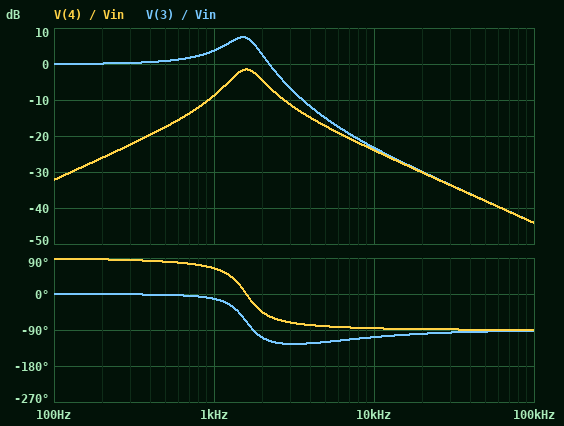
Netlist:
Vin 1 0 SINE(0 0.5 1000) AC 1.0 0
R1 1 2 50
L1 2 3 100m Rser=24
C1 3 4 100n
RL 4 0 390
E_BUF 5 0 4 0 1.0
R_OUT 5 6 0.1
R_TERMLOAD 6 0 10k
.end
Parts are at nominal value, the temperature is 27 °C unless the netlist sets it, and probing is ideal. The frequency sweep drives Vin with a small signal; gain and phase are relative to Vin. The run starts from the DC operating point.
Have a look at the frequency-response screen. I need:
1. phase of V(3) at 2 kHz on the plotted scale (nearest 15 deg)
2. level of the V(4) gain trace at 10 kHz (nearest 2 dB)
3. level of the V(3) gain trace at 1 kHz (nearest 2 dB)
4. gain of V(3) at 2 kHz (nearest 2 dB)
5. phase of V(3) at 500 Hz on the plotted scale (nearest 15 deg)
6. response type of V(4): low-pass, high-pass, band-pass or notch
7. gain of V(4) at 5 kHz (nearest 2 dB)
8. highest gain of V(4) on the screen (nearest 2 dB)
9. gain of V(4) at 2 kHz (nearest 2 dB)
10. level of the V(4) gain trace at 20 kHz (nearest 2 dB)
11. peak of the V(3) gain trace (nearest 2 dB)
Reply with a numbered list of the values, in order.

1. -105 deg
2. -24 dB
3. 4 dB
4. 2 dB
5. 0 deg
6. band-pass
7. -18 dB
8. -2 dB
9. -4 dB
10. -30 dB
11. 8 dB
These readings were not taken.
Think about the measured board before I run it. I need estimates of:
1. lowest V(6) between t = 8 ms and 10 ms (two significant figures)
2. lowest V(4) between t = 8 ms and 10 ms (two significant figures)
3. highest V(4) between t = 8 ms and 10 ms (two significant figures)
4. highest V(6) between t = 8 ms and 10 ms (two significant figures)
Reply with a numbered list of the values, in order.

1. -180 mV
2. -180 mV
3. 180 mV
4. 180 mV
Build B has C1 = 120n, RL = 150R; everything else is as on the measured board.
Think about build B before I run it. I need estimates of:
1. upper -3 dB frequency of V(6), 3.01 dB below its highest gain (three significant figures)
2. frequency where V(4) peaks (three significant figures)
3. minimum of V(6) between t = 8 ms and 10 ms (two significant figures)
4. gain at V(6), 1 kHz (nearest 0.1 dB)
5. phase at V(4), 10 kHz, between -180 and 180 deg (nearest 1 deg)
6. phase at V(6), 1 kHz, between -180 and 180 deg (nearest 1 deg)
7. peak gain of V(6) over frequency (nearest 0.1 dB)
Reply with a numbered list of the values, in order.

1. 1.64 kHz
2. 1.45 kHz
3. -100 mV
4. -13.8 dB
5. -88 deg
6. 72 deg
7. -3.5 dB
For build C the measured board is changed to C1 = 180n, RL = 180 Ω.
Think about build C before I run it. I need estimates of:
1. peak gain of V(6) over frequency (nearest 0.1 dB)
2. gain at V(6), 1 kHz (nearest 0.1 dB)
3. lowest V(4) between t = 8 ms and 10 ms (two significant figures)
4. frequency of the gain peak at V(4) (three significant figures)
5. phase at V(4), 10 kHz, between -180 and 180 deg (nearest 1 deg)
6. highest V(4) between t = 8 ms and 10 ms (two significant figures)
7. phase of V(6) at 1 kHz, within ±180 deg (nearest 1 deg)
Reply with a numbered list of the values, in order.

1. -3.0 dB
2. -6.0 dB
3. -250 mV
4. 1.19 kHz
5. -88 deg
6. 250 mV
7. 45 deg
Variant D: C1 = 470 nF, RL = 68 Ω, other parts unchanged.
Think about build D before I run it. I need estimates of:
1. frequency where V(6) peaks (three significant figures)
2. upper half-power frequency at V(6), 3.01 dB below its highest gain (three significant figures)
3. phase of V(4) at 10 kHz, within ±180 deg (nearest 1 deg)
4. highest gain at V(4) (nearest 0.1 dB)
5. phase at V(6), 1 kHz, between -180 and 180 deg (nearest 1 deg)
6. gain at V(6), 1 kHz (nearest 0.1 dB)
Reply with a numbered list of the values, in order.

1. 734 Hz
2. 856 Hz
3. -89 deg
4. -6.4 dB
5. -64 deg
6. -13.5 dB
